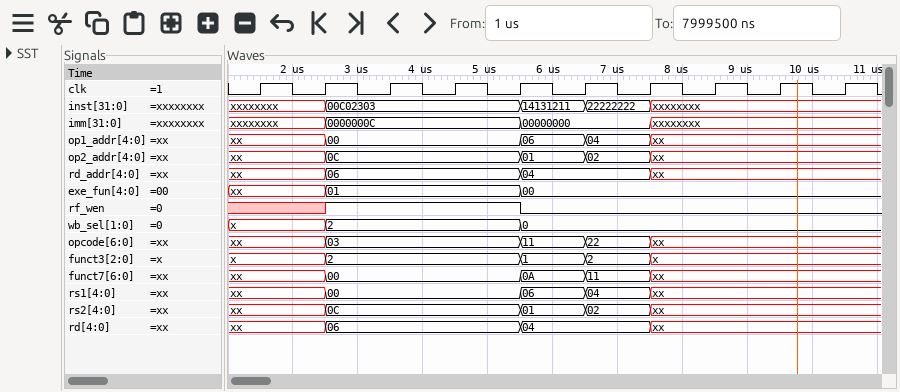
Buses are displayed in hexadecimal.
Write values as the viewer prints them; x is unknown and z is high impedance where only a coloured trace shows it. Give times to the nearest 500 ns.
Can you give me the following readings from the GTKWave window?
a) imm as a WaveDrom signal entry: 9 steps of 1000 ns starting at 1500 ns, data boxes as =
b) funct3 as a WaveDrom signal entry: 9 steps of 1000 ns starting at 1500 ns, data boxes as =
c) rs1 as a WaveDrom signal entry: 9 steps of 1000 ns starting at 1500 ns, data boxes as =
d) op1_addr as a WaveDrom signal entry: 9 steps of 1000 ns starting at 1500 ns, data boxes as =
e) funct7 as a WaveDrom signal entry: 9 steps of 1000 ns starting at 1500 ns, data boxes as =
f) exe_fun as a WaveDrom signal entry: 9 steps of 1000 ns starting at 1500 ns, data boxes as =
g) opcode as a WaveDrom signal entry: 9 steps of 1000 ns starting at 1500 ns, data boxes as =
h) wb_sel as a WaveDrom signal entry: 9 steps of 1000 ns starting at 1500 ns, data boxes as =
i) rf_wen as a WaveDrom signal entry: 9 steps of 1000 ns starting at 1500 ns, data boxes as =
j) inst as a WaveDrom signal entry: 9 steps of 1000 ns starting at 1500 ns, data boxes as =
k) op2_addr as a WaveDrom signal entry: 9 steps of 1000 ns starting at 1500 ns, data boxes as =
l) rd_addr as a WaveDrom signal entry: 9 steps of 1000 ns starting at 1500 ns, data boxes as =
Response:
{name: 'imm', wave: 'x=..=.x..', data: '0000000C 00000000'}
{name: 'funct3', wave: 'x=..==x..', data: '2 1 2'}
{name: 'rs1', wave: 'x=..==x..', data: '00 06 04'}
{name: 'op1_addr', wave: 'x=..==x..', data: '00 06 04'}
{name: 'funct7', wave: 'x=..==x..', data: '00 0A 11'}
{name: 'exe_fun', wave: 'x=..=....', data: '01 00'}
{name: 'opcode', wave: 'x=..==x..', data: '03 11 22'}
{name: 'wb_sel', wave: 'x=..=....', data: '2 0'}
{name: 'rf_wen', wave: 'x1..0....'}
{name: 'inst', wave: 'x=..==x..', data: '00C02303 14131211 22222222'}
{name: 'op2_addr', wave: 'x=..==x..', data: '0C 01 02'}
{name: 'rd_addr', wave: 'x=..=.x..', data: '06 04'}
